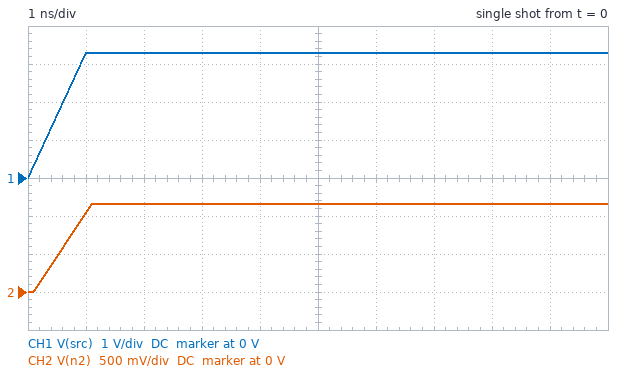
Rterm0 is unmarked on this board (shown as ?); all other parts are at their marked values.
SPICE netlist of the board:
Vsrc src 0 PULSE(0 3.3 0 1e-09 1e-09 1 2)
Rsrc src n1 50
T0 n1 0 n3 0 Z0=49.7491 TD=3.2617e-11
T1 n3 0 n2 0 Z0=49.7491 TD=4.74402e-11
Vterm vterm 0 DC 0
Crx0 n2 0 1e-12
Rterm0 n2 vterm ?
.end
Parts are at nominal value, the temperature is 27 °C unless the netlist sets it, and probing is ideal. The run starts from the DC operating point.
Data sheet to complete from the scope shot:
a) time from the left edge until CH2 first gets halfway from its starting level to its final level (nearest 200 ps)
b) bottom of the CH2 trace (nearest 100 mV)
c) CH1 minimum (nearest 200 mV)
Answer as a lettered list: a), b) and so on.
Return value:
a) 600 ps
b) 0 V
c) 0 V
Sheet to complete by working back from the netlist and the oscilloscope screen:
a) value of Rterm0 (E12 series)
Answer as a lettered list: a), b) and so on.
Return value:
a) 27 Ω
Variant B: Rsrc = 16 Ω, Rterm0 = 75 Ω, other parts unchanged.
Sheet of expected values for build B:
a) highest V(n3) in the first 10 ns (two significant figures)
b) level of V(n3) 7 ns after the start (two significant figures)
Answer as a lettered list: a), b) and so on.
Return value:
a) 2.8 V
b) 2.7 V
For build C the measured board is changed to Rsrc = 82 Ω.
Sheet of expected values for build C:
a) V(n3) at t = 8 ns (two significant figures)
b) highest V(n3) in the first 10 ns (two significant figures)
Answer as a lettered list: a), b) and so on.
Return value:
a) 820 mV
b) 840 mV
